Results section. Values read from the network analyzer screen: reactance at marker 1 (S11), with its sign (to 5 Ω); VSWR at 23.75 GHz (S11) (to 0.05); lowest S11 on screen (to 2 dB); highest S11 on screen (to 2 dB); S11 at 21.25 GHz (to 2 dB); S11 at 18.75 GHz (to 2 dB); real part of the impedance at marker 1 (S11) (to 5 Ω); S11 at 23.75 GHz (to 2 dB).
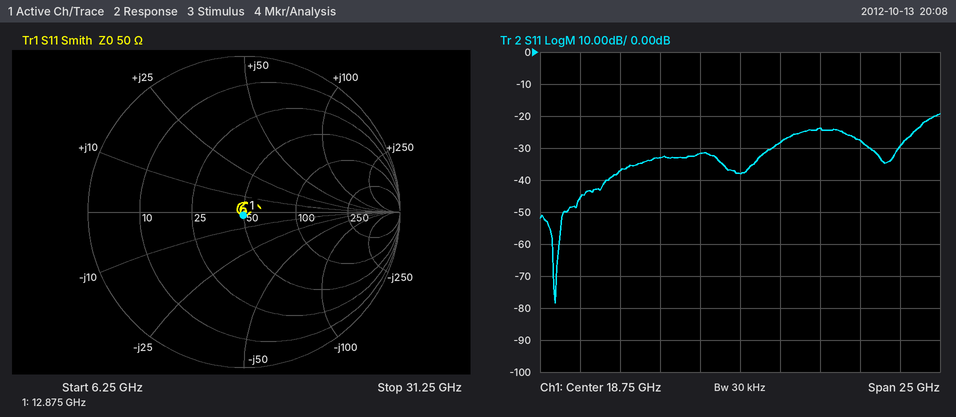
0 Ω
1.15
-78 dB
-20 dB
-28 dB
-38 dB
50 Ω
-24 dB
